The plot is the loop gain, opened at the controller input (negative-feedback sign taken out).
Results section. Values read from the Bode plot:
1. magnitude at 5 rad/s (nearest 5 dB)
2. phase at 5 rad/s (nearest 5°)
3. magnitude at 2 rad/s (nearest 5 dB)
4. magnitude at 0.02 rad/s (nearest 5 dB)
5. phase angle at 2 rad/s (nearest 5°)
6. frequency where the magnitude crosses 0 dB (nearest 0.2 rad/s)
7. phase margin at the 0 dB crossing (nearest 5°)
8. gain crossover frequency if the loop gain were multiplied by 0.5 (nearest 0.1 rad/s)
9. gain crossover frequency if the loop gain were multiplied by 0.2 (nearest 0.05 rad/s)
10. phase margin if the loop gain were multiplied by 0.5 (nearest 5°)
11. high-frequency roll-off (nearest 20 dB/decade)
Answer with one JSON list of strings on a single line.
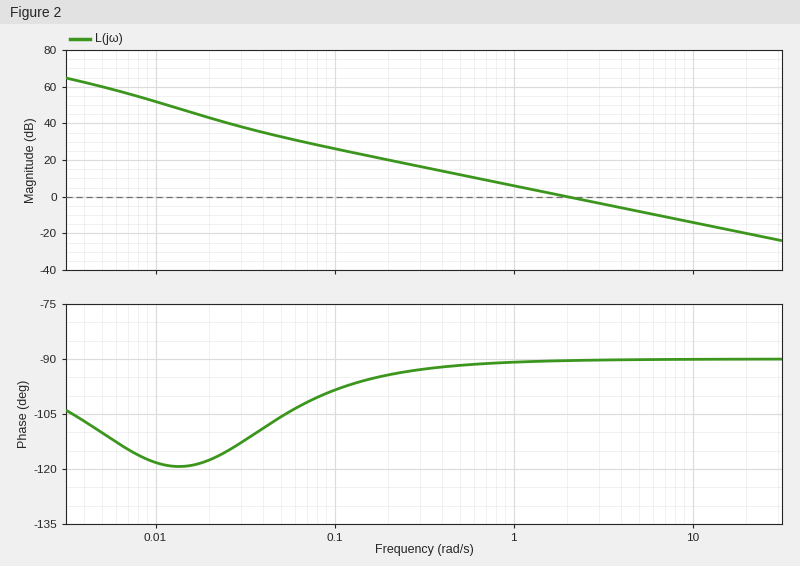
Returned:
["-10 dB", "-90°", "0 dB", "45 dB", "-90°", "2.0 rad/s", "90°", "1.0 rad/s", "0.40 rad/s", "90°", "-20 dB/decade"]
